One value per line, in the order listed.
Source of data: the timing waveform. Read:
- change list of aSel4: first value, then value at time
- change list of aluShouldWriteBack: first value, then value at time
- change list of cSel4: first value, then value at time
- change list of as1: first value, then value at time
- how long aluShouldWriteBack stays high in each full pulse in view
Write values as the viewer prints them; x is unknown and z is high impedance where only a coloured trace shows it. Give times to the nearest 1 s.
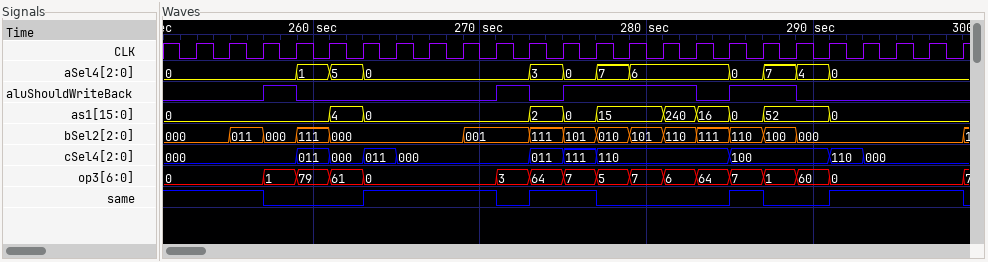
0, 1 at 259 s, 5 at 261 s, 0 at 263 s, 3 at 273 s, 0 at 275 s, 7 at 277 s, 6 at 279 s, 0 at 285 s, 7 at 287 s, 4 at 289 s, 0 at 291 s
0, 1 at 257 s, 0 at 259 s, 1 at 271 s, 0 at 273 s, 1 at 275 s, 0 at 283 s, 1 at 285 s, 0 at 289 s
000, 011 at 259 s, 000 at 261 s, 011 at 263 s, 000 at 265 s, 011 at 273 s, 111 at 275 s, 110 at 277 s, 100 at 285 s, 110 at 291 s, 000 at 293 s
0, 4 at 261 s, 0 at 263 s, 2 at 273 s, 0 at 275 s, 15 at 277 s, 240 at 281 s, 16 at 283 s, 0 at 285 s, 52 at 287 s, 0 at 291 s
2 s, 2 s, 8 s, 4 s
